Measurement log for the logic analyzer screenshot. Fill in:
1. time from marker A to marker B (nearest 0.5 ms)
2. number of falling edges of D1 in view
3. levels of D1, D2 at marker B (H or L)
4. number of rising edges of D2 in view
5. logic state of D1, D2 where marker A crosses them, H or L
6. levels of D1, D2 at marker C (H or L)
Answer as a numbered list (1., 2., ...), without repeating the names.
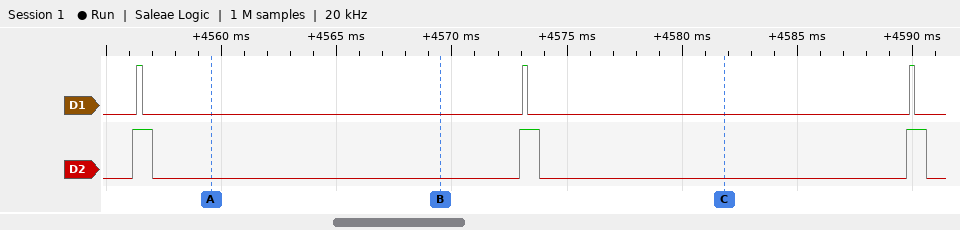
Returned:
1. 10 ms
2. 3
3. D1=L, D2=L
4. 3
5. D1=L, D2=L
6. D1=L, D2=L
